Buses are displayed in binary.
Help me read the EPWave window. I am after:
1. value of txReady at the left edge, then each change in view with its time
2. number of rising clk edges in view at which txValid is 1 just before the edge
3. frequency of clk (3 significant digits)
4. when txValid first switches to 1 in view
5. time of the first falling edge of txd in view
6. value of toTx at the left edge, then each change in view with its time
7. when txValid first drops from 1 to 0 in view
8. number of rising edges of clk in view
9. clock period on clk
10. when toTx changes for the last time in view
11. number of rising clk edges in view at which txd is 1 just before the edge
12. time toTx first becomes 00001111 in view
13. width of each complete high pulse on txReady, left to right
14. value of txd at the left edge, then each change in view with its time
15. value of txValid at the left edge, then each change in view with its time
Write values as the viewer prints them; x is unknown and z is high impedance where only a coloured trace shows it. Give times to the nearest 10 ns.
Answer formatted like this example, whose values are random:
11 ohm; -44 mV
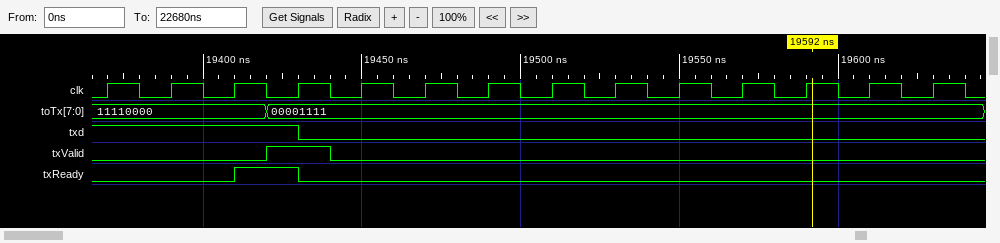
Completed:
0, 1 at 19410 ns, 0 at 19430 ns; 1; 50.0 MHz; 19420 ns; 19430 ns; 11110000, 00001111 at 19420 ns; 19440 ns; 14; 20 ns; 19420 ns; 4; 19420 ns; 20 ns; 1, 0 at 19430 ns; 0, 1 at 19420 ns, 0 at 19440 ns
